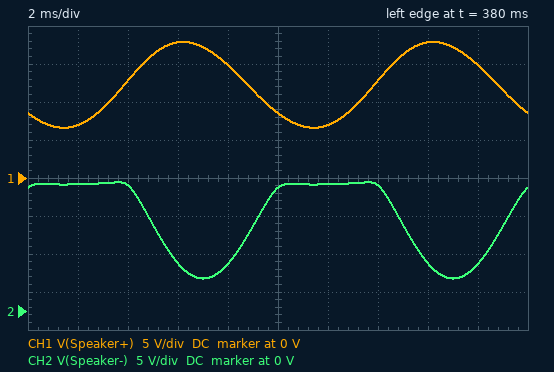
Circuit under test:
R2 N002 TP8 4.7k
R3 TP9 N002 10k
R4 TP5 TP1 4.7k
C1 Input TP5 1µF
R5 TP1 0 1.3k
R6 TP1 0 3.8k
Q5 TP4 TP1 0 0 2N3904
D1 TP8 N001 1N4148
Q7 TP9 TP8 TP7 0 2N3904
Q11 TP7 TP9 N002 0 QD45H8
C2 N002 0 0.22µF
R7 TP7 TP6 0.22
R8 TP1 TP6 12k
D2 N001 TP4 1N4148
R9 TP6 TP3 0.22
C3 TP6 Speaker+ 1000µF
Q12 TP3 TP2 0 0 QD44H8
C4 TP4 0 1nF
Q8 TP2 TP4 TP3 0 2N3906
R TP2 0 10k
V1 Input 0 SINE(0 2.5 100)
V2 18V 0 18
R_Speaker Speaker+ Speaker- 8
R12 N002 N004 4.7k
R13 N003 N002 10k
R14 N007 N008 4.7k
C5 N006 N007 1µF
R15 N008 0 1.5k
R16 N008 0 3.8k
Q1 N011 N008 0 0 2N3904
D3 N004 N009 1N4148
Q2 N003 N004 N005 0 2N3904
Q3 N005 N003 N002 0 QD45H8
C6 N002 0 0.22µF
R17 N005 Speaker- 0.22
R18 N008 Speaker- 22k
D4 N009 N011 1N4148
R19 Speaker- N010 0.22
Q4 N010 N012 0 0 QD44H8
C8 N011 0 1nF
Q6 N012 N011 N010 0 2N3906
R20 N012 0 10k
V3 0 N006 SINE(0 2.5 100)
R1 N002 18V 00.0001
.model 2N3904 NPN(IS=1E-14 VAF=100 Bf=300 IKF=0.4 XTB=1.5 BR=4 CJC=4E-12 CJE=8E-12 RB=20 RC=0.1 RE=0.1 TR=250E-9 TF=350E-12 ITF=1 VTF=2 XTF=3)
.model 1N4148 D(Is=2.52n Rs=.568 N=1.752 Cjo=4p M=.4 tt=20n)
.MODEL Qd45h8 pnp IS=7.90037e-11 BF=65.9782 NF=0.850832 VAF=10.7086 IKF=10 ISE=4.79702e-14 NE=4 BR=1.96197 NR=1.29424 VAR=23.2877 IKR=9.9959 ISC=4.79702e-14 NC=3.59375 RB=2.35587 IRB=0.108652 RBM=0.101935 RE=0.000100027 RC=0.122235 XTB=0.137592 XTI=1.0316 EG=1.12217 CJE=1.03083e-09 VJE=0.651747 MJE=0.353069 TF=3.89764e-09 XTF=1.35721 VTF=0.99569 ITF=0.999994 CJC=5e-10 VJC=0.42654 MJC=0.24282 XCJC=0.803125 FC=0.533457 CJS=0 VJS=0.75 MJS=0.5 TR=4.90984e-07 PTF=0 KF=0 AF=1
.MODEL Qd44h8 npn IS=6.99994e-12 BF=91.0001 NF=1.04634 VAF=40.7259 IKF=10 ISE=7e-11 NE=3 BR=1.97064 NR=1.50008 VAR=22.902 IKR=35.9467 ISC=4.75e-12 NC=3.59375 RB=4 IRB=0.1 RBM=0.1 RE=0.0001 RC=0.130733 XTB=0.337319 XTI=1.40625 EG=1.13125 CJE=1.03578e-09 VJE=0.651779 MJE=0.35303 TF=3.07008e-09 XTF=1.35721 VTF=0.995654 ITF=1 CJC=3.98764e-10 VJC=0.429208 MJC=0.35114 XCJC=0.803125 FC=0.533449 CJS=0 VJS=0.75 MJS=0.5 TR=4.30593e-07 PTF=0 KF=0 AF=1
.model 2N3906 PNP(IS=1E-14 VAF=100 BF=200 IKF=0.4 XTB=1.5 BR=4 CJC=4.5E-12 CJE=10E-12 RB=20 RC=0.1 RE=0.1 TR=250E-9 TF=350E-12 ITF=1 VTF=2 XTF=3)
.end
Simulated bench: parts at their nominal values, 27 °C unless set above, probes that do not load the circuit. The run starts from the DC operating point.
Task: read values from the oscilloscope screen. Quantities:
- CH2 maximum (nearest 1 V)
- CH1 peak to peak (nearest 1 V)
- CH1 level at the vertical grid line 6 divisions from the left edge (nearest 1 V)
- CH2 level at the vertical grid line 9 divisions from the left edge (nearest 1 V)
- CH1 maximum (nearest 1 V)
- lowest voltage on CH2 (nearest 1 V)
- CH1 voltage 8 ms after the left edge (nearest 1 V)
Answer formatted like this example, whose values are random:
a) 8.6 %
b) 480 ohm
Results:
a) 17 V
b) 11 V
c) 7 V
d) 6 V
e) 18 V
f) 4 V
g) 15 V
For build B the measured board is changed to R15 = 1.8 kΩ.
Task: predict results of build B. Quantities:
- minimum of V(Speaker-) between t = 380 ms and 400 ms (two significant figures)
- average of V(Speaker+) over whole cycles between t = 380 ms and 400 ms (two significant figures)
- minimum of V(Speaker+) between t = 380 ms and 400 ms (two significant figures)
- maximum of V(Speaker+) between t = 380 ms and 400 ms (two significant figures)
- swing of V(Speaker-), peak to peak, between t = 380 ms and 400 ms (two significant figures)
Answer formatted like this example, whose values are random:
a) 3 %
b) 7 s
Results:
a) 2.6 V
b) 11 V
c) 5.6 V
d) 17 V
e) 14 V
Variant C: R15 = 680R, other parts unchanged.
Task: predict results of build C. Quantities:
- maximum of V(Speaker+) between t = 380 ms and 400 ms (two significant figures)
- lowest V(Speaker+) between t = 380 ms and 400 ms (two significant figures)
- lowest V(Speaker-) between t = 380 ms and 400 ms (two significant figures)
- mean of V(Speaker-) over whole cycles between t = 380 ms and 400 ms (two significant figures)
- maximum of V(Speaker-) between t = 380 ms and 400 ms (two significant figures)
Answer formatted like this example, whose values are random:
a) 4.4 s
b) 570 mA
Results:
a) 22 V
b) 11 V
c) 15 V
d) 17 V
e) 18 V
